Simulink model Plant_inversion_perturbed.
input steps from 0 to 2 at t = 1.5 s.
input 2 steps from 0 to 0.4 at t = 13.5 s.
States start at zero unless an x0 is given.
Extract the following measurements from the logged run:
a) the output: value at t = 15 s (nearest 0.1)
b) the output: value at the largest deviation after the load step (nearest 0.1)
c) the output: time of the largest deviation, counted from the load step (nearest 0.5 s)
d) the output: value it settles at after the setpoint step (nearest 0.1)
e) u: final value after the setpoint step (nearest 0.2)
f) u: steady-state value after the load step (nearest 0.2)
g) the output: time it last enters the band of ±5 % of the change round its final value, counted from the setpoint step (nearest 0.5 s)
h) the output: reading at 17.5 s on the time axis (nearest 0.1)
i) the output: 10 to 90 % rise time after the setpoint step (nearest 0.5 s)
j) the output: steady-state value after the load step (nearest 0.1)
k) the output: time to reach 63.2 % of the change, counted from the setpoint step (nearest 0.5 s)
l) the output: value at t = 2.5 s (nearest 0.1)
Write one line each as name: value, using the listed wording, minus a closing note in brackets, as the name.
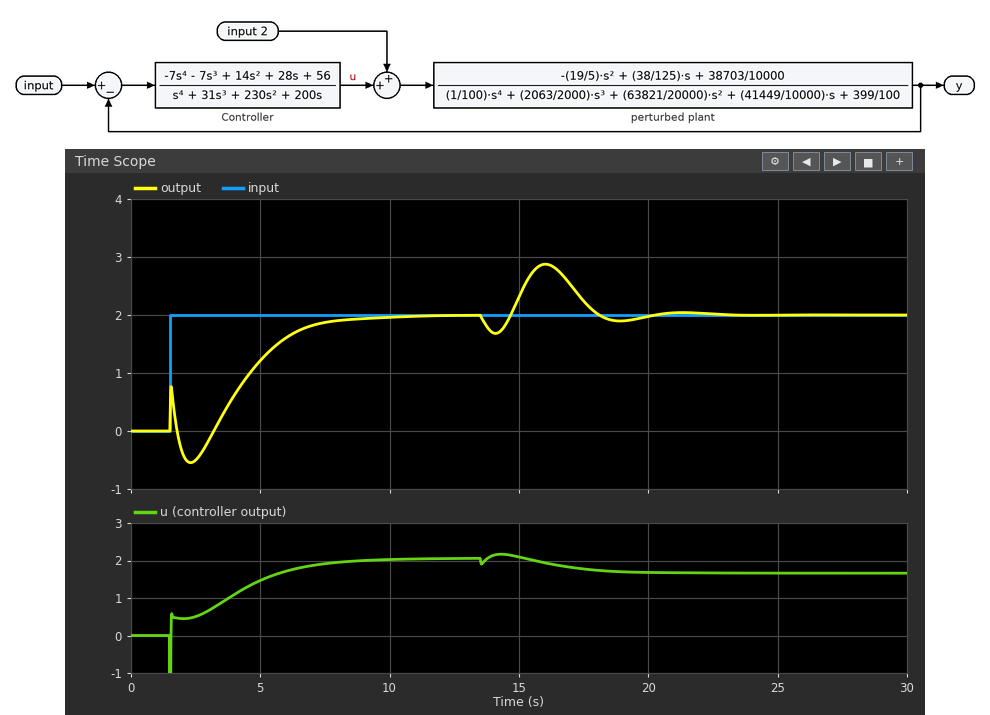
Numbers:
the output: value at t = 15 s: 2.3
the output: value at the largest deviation after the load step: 2.9
the output: time of the largest deviation, counted from the load step: 2.5 s
the output: value it settles at after the setpoint step: 2.0
u: final value after the setpoint step: 2.0
u: steady-state value after the load step: 1.6
the output: time it last enters the band of ±5 % of the change round its final value, counted from the setpoint step: 6.5 s
the output: reading at 17.5 s on the time axis: 2.2
the output: 10 to 90 % rise time after the setpoint step: 5.5 s
the output: steady-state value after the load step: 2.0
the output: time to reach 63.2 % of the change, counted from the setpoint step: 3.5 s
the output: value at t = 2.5 s: -0.5
